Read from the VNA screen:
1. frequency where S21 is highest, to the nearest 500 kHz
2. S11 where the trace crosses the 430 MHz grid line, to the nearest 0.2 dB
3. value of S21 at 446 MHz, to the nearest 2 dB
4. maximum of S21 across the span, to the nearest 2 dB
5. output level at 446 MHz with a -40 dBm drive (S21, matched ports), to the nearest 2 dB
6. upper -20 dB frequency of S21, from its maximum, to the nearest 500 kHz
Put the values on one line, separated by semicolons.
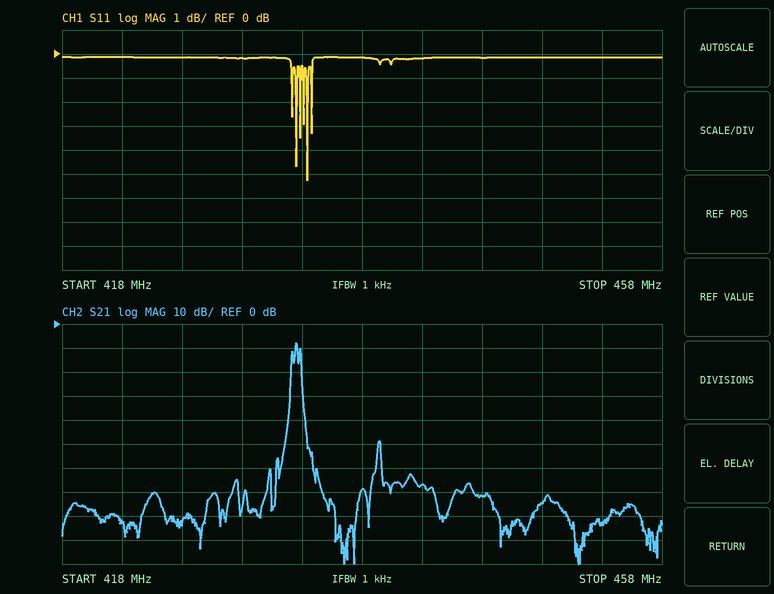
433.5 MHz; -0.2 dB; -72 dB; -8 dB; -112 dBm; 434.0 MHz
